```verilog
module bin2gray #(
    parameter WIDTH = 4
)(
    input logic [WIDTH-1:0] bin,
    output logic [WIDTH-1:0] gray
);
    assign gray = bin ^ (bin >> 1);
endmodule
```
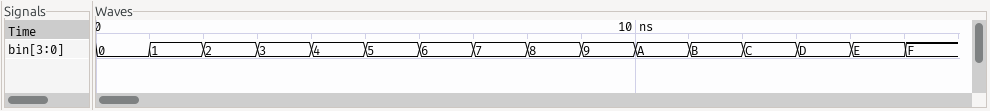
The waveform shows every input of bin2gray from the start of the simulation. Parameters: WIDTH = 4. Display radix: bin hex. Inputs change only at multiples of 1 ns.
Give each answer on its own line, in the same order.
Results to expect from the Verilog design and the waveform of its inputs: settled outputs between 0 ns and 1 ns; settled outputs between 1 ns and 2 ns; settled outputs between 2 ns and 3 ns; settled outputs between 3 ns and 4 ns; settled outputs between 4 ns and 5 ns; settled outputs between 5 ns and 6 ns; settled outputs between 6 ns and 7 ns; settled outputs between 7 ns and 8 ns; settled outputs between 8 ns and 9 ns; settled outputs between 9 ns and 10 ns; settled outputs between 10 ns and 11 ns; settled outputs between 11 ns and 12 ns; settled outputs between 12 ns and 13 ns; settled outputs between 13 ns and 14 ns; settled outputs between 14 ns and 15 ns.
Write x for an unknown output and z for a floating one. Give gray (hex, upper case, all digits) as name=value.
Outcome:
gray=0
gray=1
gray=3
gray=2
gray=6
gray=7
gray=5
gray=4
gray=C
gray=D
gray=F
gray=E
gray=A
gray=B
gray=9
